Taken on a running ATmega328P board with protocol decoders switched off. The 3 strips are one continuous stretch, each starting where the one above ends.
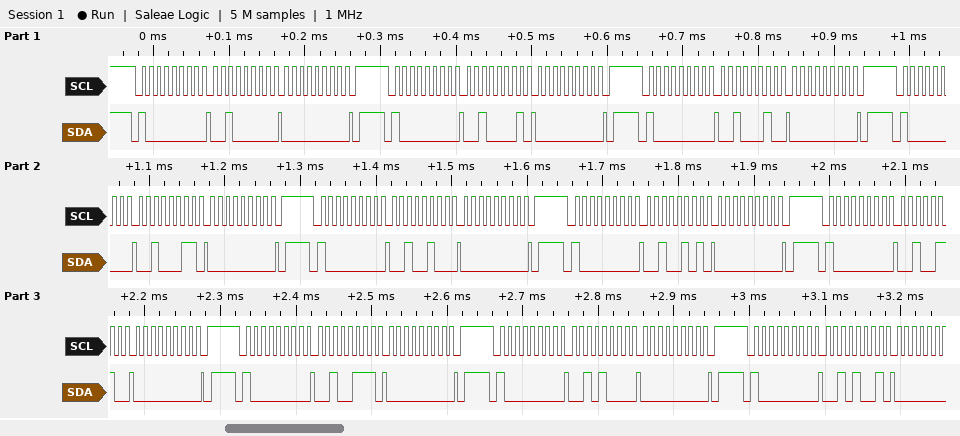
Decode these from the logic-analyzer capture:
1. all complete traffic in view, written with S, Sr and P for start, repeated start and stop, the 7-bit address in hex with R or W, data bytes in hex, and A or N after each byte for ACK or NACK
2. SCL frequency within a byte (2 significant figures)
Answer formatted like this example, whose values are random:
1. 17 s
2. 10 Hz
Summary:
1. S 40W A 20 A 00 A P S 40W A 21 A 00 A P S 40W A 22 A 00 A P S 40W A 23 A 00 A P S 40W A 24 A 00 A P S 40W A 25 A 00 A P S 40W A 26 A 00 A P S 40W A 27 A 00 A P S 40W A 28 A 00 A P S 40W A 29 A
2. 100 kHz
